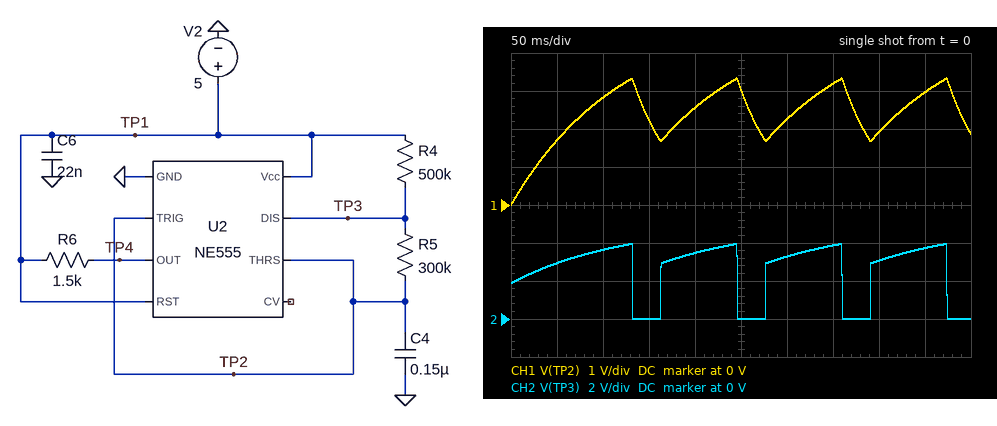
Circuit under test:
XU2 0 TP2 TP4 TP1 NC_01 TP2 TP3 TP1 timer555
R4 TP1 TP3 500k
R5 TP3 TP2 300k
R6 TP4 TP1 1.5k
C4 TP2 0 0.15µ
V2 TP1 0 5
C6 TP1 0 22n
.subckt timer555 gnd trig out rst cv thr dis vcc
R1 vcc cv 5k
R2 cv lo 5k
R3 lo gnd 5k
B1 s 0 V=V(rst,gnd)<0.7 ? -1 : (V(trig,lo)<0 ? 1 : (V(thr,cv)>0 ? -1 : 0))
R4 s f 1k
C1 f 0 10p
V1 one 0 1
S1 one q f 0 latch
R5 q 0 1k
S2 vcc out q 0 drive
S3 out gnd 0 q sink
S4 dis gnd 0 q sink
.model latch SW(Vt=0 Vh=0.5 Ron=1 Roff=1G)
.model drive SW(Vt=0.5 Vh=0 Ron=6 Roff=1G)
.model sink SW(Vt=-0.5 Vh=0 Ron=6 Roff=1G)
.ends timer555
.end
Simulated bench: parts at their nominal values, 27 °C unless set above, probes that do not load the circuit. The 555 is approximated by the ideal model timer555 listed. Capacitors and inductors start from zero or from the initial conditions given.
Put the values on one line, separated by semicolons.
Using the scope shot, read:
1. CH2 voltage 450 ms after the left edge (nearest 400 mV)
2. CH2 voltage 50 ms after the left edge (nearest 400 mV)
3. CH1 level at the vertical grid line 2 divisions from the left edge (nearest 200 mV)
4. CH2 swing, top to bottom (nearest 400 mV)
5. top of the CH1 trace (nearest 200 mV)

3.6 V; 2.8 V; 2.8 V; 4.0 V; 3.4 V
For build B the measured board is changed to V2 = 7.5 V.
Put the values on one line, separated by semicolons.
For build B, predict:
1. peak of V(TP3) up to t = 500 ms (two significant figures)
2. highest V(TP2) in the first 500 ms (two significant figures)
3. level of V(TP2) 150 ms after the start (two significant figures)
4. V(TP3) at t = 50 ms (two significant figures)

5.9 V; 5.0 V; 3.3 V; 4.4 V
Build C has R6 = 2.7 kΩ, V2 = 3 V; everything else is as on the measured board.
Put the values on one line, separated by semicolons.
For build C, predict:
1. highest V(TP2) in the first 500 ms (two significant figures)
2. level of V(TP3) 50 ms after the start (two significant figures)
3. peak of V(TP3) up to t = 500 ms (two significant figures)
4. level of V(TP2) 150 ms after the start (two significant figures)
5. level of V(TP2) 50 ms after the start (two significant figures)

2.0 V; 1.8 V; 2.4 V; 1.3 V; 1.0 V
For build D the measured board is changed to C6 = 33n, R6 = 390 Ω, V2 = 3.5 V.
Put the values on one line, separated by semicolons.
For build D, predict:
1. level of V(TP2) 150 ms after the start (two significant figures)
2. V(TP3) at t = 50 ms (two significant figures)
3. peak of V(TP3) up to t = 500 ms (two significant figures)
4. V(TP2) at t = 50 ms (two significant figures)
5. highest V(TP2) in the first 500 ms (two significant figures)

1.6 V; 2.1 V; 2.8 V; 1.2 V; 2.3 V
